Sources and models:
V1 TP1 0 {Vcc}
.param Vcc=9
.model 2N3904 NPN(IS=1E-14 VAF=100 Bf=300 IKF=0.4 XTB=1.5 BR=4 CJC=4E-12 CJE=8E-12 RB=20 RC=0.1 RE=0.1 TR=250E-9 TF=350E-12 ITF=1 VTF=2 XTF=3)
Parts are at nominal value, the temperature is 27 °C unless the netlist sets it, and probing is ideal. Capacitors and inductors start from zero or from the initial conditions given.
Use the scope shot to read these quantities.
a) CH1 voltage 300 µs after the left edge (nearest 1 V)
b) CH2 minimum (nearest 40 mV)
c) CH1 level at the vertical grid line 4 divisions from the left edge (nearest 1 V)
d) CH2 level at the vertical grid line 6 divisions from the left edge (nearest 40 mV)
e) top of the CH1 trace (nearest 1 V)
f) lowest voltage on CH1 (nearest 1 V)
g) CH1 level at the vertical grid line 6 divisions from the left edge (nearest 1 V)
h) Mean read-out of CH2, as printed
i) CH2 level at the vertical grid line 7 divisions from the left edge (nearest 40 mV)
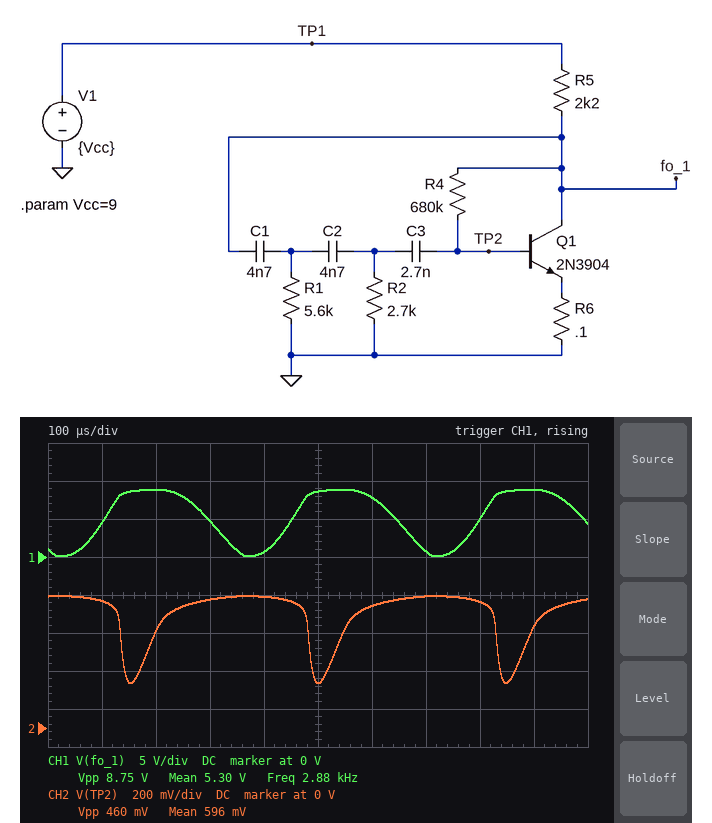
5 V
240 mV
1 V
640 mV
9 V
0 V
8 V
596 mV
680 mV
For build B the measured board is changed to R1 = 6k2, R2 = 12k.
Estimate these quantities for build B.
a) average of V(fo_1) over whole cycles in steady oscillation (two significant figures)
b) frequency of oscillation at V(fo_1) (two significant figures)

5.0 V
1.7 kHz
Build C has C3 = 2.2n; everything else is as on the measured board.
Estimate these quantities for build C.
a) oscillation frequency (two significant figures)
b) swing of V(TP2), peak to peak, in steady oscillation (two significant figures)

3.1 kHz
470 mV
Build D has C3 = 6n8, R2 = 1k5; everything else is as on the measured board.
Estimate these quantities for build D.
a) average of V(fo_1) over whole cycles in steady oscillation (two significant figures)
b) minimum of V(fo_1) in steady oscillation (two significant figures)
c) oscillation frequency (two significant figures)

5.0 V
110 mV
2.5 kHz
